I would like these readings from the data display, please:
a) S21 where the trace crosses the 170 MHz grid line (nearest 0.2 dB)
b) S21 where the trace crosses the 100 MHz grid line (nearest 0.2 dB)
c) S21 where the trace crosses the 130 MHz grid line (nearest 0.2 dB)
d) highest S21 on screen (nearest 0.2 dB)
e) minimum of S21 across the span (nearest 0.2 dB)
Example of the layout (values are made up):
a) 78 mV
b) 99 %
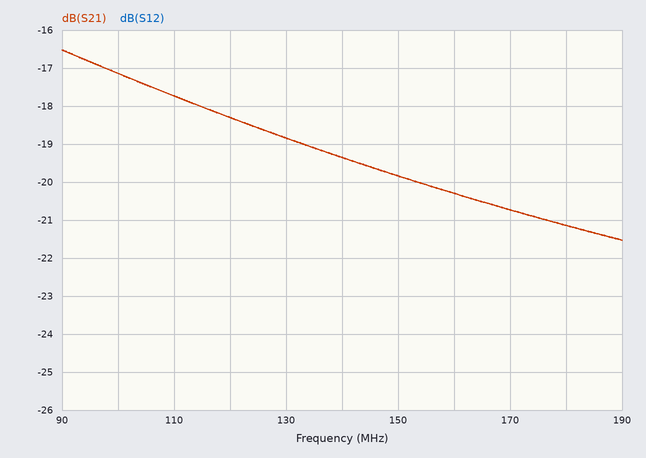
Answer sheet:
a) -20.8 dB
b) -17.2 dB
c) -18.8 dB
d) -16.6 dB
e) -21.6 dB
